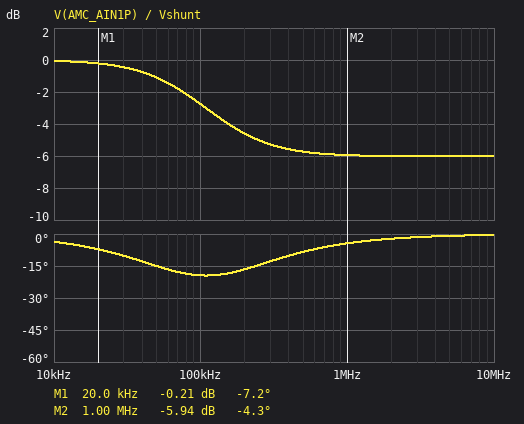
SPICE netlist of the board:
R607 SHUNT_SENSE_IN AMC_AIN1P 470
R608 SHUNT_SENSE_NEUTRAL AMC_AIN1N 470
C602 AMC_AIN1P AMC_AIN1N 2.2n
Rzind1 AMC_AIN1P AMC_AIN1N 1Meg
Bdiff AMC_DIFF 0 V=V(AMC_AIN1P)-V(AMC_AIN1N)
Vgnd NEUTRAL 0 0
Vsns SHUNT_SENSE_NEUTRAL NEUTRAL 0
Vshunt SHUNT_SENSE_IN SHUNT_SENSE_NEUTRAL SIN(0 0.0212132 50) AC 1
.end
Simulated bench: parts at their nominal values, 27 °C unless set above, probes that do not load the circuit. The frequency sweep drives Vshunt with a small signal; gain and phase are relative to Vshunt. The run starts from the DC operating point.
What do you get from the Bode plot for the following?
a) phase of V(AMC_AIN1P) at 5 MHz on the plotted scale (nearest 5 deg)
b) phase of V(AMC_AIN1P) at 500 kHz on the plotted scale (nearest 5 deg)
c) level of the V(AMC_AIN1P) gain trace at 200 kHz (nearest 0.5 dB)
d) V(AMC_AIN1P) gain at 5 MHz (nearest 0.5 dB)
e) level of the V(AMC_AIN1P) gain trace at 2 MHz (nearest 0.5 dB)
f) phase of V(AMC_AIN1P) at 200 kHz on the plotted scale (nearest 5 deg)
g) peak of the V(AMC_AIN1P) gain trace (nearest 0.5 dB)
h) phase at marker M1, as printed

0 deg
-10 deg
-4.5 dB
-6.0 dB
-6.0 dB
-15 deg
0 dB
-7.2 deg
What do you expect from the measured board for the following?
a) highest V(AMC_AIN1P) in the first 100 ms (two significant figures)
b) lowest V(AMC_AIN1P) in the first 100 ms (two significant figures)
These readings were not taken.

21 mV
-21 mV
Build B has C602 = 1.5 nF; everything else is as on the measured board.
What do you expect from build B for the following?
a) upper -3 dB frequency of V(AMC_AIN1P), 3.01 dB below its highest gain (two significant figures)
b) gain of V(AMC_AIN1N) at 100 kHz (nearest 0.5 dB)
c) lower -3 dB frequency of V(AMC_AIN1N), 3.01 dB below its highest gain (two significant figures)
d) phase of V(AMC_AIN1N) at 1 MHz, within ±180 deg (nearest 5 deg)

160 kHz
-9.5 dB
110 kHz
5 deg
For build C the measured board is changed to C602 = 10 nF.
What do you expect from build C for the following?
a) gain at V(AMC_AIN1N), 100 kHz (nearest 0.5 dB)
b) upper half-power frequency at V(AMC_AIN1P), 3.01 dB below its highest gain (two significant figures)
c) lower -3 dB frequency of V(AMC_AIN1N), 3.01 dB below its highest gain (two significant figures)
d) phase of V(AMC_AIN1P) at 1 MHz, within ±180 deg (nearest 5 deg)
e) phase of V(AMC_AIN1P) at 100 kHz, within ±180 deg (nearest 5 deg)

-6.0 dB
24 kHz
17 kHz
0 deg
-10 deg
